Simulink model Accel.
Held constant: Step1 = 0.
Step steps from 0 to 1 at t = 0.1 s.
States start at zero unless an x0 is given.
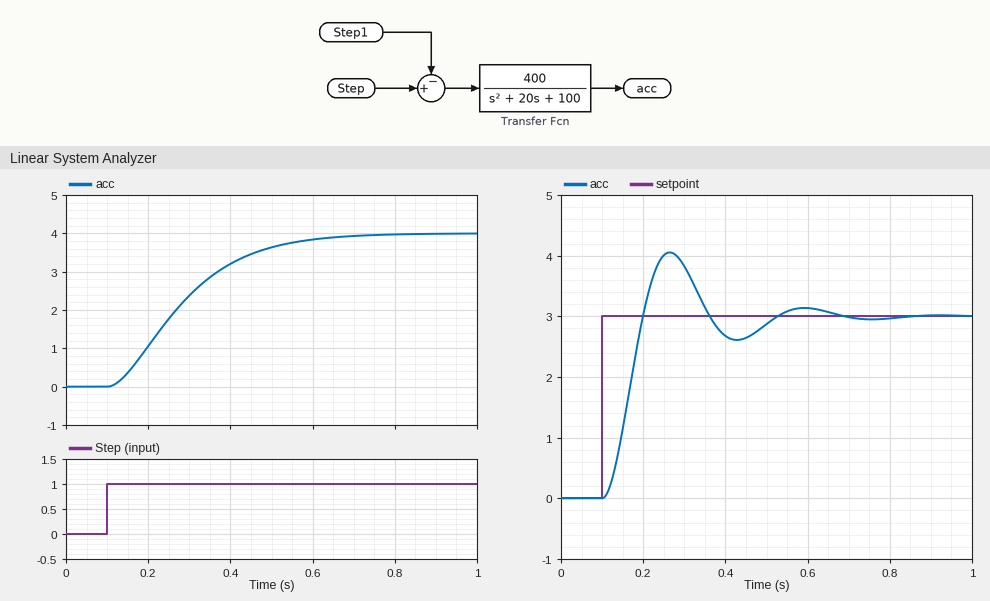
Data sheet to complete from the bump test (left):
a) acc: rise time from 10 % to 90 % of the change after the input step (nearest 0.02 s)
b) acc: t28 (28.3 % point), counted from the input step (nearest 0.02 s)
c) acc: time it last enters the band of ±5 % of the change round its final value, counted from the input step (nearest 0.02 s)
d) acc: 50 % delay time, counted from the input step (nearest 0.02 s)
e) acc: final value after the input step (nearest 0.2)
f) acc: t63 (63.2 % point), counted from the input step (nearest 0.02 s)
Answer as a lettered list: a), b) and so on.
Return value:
a) 0.34 s
b) 0.10 s
c) 0.48 s
d) 0.16 s
e) 4.0
f) 0.22 s
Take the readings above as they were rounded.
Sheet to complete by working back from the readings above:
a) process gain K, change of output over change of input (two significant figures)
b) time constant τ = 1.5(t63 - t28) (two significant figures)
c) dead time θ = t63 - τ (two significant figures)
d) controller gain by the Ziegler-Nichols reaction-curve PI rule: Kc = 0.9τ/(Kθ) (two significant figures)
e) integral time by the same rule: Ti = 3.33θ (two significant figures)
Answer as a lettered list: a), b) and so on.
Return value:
a) 4.0
b) 0.18 s
c) 0.040 s
d) 1.0
e) 0.13 s
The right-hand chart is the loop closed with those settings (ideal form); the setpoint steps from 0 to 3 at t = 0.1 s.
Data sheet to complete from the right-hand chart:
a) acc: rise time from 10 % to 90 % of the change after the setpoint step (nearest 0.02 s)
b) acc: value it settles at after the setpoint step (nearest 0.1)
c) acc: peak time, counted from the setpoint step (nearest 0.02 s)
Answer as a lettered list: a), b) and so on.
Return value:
a) 0.06 s
b) 3.0
c) 0.16 s
